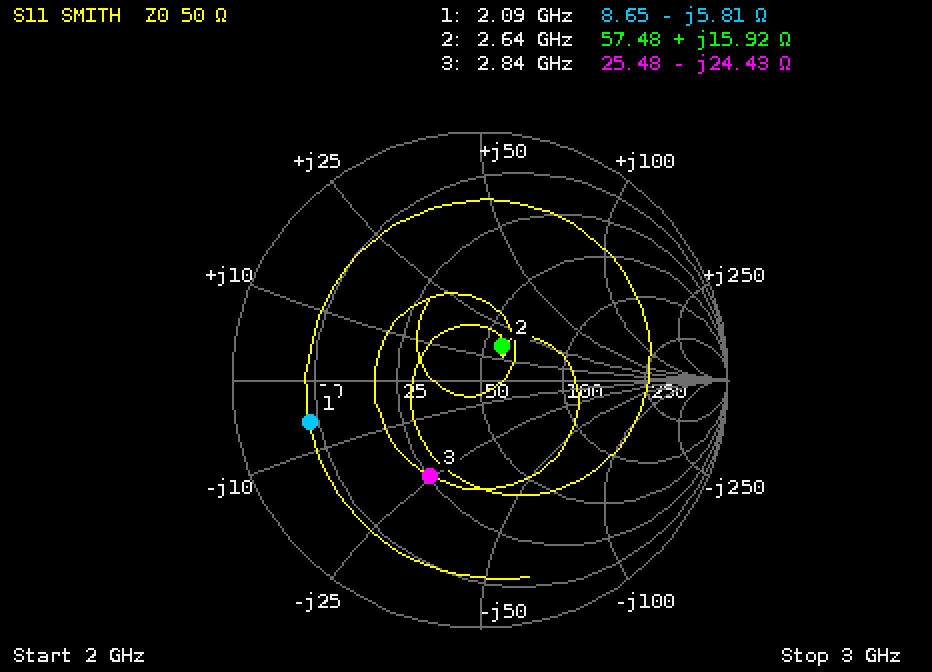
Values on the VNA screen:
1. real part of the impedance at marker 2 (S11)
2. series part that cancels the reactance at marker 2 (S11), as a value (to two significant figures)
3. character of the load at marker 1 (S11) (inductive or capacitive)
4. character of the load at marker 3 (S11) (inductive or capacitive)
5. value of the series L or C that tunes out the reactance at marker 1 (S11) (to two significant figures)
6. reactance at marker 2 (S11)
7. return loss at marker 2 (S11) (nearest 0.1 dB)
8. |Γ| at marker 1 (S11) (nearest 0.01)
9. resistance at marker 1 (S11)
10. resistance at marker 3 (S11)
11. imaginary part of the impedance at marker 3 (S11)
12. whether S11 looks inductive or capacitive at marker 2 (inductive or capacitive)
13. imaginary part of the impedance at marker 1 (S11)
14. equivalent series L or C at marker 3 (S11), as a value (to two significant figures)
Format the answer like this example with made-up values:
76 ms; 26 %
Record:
57.48 Ω; 3.8 pF; capacitive; capacitive; 440 pH; +15.92 Ω; 15.8 dB; 0.71; 8.65 Ω; 25.48 Ω; -24.43 Ω; inductive; -5.81 Ω; 2.3 pF
